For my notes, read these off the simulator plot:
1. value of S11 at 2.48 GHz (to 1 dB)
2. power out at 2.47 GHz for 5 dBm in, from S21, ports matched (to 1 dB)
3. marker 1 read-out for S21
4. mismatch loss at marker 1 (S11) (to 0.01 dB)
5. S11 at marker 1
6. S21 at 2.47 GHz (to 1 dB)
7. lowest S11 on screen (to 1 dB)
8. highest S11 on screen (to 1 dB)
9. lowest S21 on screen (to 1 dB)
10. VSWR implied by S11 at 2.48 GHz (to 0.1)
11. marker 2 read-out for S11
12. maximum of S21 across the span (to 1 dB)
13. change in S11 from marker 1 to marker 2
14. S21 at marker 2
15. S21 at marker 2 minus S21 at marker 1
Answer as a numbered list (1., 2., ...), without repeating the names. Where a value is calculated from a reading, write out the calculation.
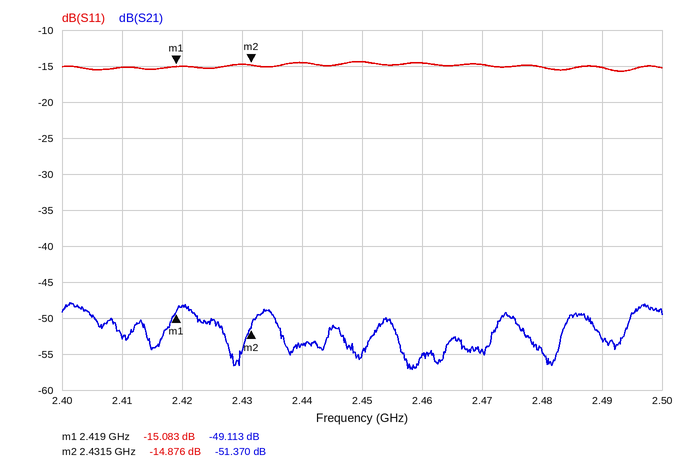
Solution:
1. -15 dB
2. 5 dBm + (-54 dB) = -49 dBm
3. -49.113 dB
4. −10 log10(1 − 10^(-15.083/10)) ≈ 0.14 dB
5. -15.083 dB
6. -54 dB
7. -16 dB
8. -14 dB
9. -57 dB
10. |Γ| = 10^(-15/20) = 0.1778; VSWR = (1 + 0.1778)/(1 − 0.1778) ≈ 1.4
11. -14.876 dB
12. -48 dB
13. -14.876 − (-15.083) = 0.207 dB
14. -51.370 dB
15. -51.37 − (-49.113) = -2.257 dB
